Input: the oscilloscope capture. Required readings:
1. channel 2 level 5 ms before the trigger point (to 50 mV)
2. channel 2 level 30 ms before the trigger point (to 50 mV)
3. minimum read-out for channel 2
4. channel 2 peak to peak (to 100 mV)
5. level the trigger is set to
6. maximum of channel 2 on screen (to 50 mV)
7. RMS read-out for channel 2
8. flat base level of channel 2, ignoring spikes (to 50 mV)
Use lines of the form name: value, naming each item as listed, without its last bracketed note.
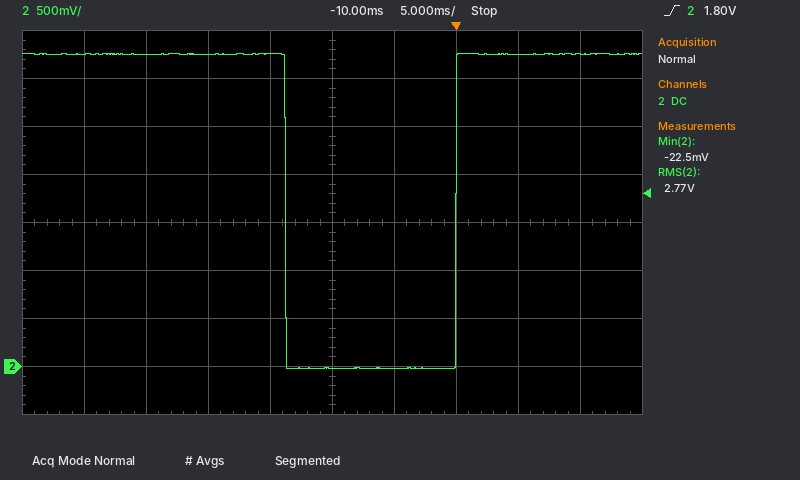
channel 2 level 5 ms before the trigger point: 0 mV
channel 2 level 30 ms before the trigger point: 3.25 V
minimum read-out for channel 2: -22.5 mV
channel 2 peak to peak: 3.30 V
level the trigger is set to: 1.80 V
maximum of channel 2 on screen: 3.25 V
RMS read-out for channel 2: 2.77 V
flat base level of channel 2, ignoring spikes: 0 mV
